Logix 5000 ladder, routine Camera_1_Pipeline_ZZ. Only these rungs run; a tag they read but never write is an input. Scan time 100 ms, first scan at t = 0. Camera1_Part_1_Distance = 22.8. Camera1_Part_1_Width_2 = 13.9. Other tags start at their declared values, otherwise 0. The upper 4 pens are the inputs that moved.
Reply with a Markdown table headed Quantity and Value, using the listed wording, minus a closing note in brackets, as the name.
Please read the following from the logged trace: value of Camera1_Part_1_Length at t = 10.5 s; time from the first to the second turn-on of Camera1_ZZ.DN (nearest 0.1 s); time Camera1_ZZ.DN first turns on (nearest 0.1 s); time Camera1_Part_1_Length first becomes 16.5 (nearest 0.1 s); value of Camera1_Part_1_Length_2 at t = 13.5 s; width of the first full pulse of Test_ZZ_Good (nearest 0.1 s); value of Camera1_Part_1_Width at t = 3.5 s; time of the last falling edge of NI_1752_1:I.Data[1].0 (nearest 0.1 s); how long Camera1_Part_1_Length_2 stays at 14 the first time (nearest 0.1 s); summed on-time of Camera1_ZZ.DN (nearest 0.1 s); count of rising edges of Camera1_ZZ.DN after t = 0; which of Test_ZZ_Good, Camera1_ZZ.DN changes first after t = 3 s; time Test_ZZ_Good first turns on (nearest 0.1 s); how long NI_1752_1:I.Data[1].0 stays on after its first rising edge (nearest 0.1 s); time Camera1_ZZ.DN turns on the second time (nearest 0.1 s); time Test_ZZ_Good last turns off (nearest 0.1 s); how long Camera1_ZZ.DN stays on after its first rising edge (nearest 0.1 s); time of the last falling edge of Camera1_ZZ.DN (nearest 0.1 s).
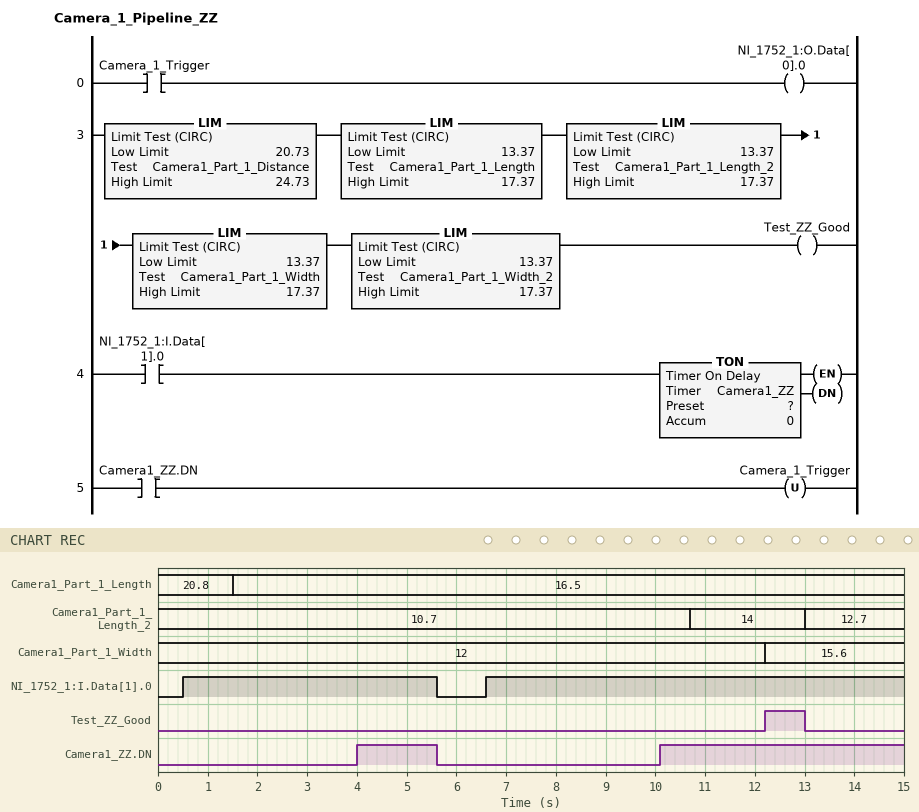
| Quantity | Value |
|---|---|
| value of Camera1_Part_1_Length at t = 10.5 s | 16.5 |
| time from the first to the second turn-on of Camera1_ZZ.DN | 6.1 s |
| time Camera1_ZZ.DN first turns on | 4.0 s |
| time Camera1_Part_1_Length first becomes 16.5 | 1.5 s |
| value of Camera1_Part_1_Length_2 at t = 13.5 s | 12.7 |
| width of the first full pulse of Test_ZZ_Good | 0.8 s |
| value of Camera1_Part_1_Width at t = 3.5 s | 12 |
| time of the last falling edge of NI_1752_1:I.Data[1].0 | 5.6 s |
| how long Camera1_Part_1_Length_2 stays at 14 the first time | 2.3 s |
| summed on-time of Camera1_ZZ.DN | 6.5 s |
| count of rising edges of Camera1_ZZ.DN after t = 0 | 2 |
| which of Test_ZZ_Good, Camera1_ZZ.DN changes first after t = 3 s | Camera1_ZZ.DN |
| time Test_ZZ_Good first turns on | 12.2 s |
| how long NI_1752_1:I.Data[1].0 stays on after its first rising edge | 5.1 s |
| time Camera1_ZZ.DN turns on the second time | 10.1 s |
| time Test_ZZ_Good last turns off | 13.0 s |
| how long Camera1_ZZ.DN stays on after its first rising edge | 1.6 s |
| time of the last falling edge of Camera1_ZZ.DN | 5.6 s |
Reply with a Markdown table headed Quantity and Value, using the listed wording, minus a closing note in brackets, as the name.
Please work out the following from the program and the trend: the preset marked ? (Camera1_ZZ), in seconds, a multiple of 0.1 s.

| Quantity | Value |
|---|---|
| the preset marked ? (Camera1_ZZ), in seconds, a multiple of 0.1 s | 3.5 s |
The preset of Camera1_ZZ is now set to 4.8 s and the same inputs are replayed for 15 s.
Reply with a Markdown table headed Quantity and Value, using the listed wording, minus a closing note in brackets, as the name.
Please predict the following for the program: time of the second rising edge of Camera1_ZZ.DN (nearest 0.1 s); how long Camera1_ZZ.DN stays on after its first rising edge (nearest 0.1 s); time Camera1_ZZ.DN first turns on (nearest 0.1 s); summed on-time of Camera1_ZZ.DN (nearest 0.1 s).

| Quantity | Value |
|---|---|
| time of the second rising edge of Camera1_ZZ.DN | 11.4 s |
| how long Camera1_ZZ.DN stays on after its first rising edge | 0.3 s |
| time Camera1_ZZ.DN first turns on | 5.3 s |
| summed on-time of Camera1_ZZ.DN | 3.9 s |
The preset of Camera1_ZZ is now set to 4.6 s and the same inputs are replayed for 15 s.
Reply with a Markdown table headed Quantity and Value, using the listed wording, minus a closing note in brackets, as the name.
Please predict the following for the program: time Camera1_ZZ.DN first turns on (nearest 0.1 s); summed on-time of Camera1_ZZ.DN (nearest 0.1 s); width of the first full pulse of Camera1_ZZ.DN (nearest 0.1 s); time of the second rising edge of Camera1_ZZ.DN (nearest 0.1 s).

| Quantity | Value |
|---|---|
| time Camera1_ZZ.DN first turns on | 5.1 s |
| summed on-time of Camera1_ZZ.DN | 4.3 s |
| width of the first full pulse of Camera1_ZZ.DN | 0.5 s |
| time of the second rising edge of Camera1_ZZ.DN | 11.2 s |
